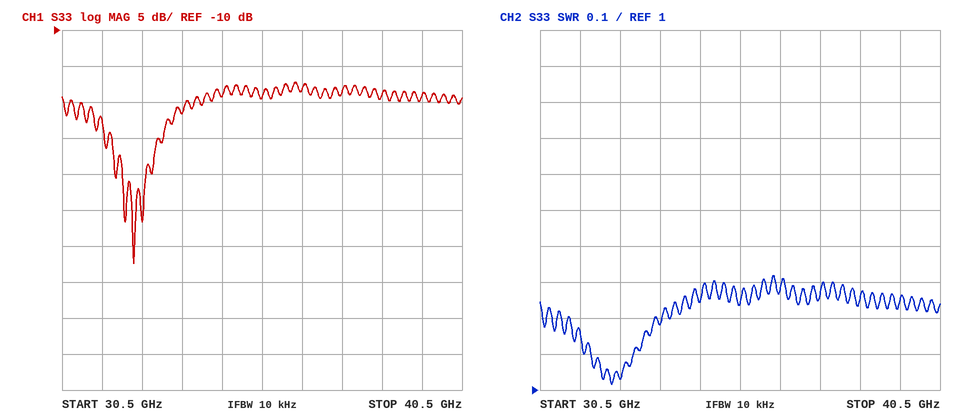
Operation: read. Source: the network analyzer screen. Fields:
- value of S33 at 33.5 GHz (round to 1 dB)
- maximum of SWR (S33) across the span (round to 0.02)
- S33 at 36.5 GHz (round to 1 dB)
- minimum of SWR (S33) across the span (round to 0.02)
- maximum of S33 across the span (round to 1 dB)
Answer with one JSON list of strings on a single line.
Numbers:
["-22 dB", "1.32", "-18 dB", "1.02", "-17 dB"]
